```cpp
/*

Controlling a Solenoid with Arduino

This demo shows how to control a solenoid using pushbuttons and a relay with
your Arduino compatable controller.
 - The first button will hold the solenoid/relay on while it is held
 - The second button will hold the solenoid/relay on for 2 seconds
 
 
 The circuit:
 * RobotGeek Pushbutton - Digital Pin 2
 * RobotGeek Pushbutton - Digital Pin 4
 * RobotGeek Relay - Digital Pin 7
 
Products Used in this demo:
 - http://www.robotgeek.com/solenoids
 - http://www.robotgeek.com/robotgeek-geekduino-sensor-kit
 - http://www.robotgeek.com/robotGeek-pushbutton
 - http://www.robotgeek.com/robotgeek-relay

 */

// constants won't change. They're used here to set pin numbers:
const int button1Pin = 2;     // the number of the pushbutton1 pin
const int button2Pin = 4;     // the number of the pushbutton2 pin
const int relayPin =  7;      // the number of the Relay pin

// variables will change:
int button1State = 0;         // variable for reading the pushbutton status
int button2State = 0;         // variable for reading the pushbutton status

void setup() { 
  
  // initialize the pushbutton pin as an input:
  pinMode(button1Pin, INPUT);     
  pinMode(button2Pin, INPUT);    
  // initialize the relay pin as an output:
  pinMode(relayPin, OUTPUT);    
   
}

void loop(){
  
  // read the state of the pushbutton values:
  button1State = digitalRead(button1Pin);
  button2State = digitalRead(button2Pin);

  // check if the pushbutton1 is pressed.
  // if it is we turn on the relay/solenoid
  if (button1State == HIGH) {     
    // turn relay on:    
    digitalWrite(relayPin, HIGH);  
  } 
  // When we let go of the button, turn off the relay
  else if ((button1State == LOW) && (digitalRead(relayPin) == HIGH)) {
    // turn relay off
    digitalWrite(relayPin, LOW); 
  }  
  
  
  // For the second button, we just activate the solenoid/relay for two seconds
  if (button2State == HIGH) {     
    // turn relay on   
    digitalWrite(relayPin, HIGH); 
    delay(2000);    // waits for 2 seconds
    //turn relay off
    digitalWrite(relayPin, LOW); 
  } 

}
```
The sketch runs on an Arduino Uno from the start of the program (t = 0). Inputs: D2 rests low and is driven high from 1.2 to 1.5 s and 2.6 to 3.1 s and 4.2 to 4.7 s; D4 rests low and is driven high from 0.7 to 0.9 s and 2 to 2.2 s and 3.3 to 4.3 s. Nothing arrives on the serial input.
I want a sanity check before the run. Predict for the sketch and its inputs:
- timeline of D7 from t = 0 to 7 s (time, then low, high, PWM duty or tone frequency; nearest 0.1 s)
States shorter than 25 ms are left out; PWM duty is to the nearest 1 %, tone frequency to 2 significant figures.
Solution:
0 s low; 0.7 s high; 3.1 s low; 3.3 s high; 5.3 s low
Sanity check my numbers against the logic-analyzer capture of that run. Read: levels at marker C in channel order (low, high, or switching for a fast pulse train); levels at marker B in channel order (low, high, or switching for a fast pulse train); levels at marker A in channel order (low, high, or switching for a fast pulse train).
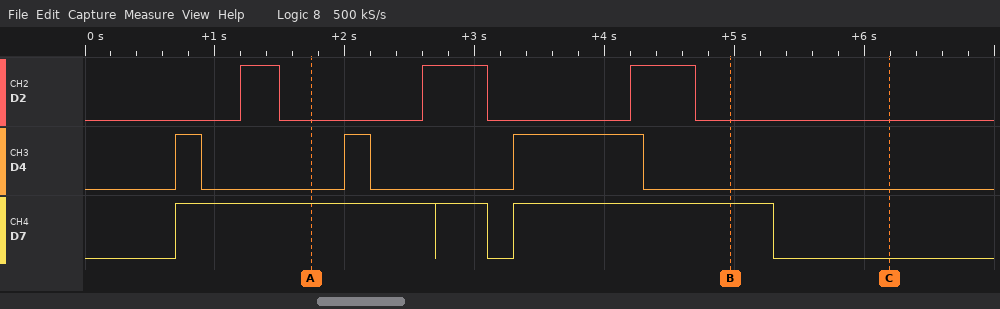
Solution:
D2 low, D4 low, D7 low
D2 low, D4 low, D7 high
D2 low, D4 low, D7 high
